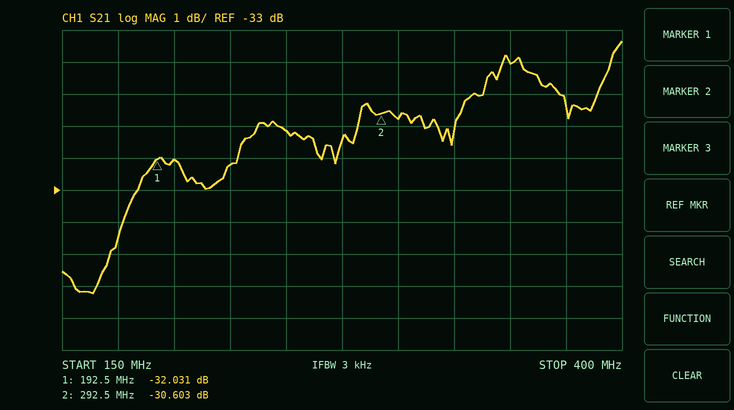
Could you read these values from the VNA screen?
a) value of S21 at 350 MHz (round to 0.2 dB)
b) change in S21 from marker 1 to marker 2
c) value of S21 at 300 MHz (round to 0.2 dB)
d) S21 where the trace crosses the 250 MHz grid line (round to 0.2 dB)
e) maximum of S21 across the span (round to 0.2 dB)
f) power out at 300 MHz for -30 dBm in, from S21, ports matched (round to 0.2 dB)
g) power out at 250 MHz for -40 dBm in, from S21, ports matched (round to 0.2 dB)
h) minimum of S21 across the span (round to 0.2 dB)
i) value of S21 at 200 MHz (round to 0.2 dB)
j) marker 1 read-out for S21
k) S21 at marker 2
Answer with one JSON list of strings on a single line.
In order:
["-29.0 dB", "1.428 dB", "-30.8 dB", "-31.2 dB", "-28.4 dB", "-60.8 dBm", "-71.2 dBm", "-36.2 dB", "-32.0 dB", "-32.031 dB", "-30.603 dB"]
